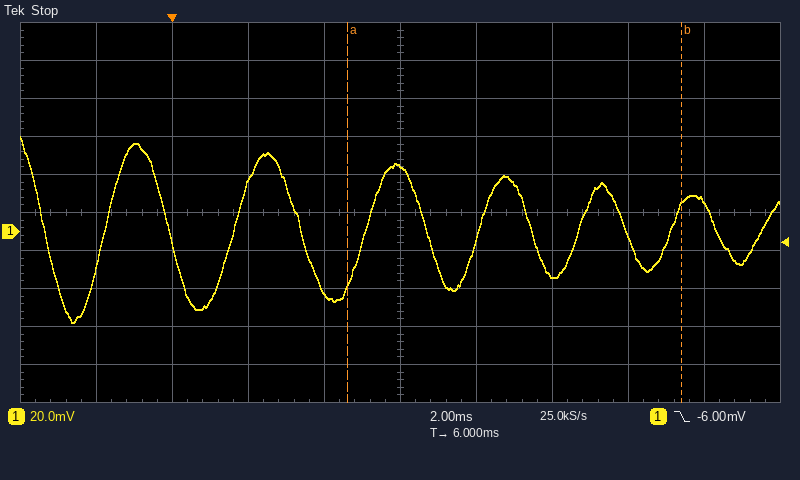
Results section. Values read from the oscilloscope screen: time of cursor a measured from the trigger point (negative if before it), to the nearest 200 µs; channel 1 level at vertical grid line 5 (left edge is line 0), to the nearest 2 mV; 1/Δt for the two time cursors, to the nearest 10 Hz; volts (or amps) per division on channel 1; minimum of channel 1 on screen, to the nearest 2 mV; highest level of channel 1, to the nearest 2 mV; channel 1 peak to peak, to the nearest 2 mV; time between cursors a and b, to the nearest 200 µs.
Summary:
+4.6 ms
34 mV
110 Hz
20 mV
-48 mV
50 mV
98 mV
8.8 ms
